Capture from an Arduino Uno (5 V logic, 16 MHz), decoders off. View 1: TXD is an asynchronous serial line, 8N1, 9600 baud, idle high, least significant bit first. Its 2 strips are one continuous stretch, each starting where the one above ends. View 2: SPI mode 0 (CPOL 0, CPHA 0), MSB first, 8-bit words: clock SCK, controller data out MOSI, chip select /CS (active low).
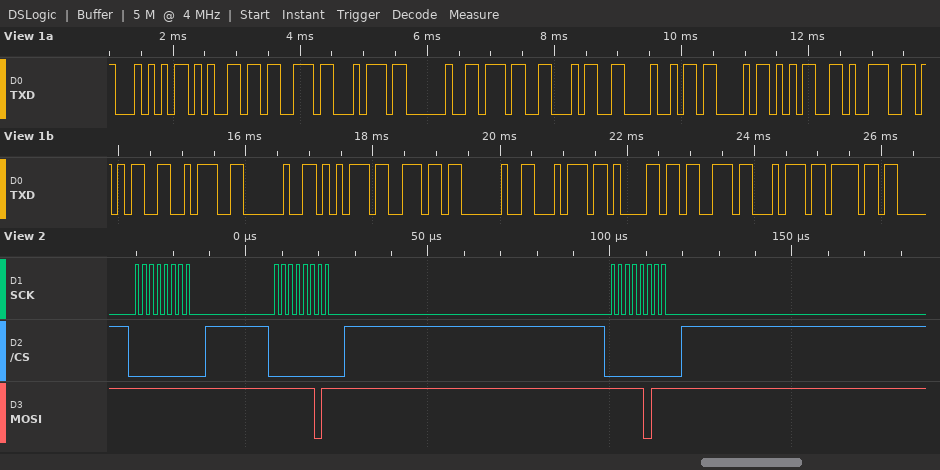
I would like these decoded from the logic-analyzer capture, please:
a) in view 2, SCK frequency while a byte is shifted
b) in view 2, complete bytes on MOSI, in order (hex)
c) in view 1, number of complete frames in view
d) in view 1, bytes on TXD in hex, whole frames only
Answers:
500 kHz
FF FD FB
22
54 65 73 74 20 37 34 48 43 35 39 35 3A 20 75 6E 20 74 61 73 74 6F
